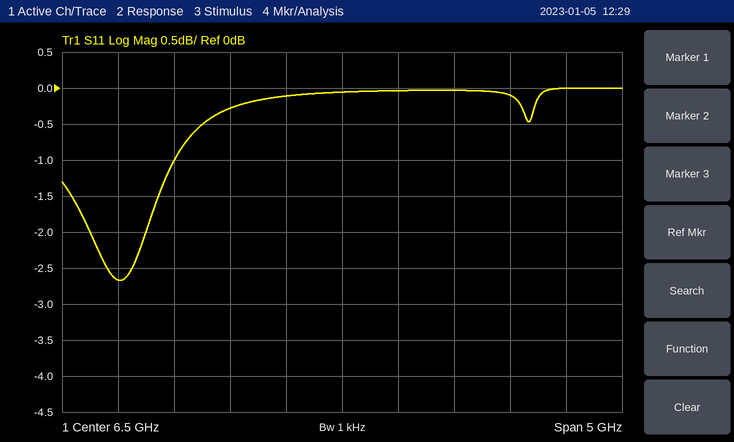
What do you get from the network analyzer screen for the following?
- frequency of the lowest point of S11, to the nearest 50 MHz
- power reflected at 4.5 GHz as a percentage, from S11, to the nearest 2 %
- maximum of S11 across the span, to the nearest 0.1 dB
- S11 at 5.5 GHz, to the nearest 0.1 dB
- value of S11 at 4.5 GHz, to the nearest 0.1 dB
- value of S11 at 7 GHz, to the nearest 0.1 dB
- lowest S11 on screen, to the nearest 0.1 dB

4.50 GHz
54 %
0.0 dB
-0.3 dB
-2.7 dB
0.0 dB
-2.7 dB
